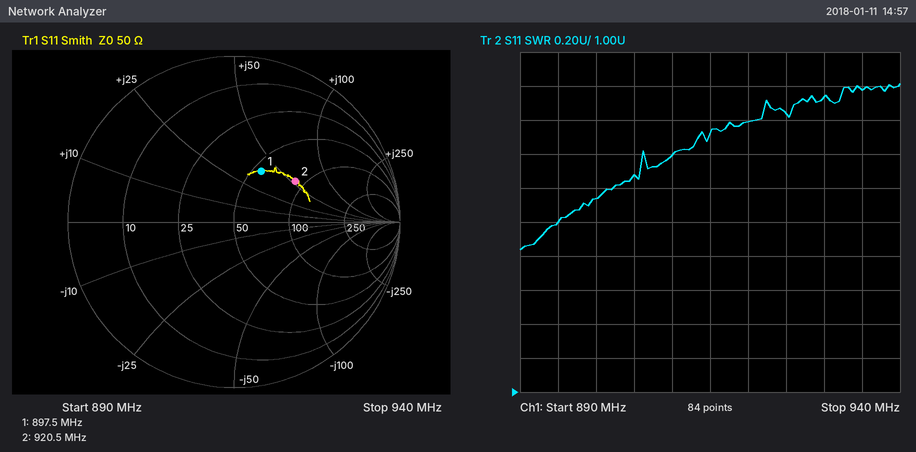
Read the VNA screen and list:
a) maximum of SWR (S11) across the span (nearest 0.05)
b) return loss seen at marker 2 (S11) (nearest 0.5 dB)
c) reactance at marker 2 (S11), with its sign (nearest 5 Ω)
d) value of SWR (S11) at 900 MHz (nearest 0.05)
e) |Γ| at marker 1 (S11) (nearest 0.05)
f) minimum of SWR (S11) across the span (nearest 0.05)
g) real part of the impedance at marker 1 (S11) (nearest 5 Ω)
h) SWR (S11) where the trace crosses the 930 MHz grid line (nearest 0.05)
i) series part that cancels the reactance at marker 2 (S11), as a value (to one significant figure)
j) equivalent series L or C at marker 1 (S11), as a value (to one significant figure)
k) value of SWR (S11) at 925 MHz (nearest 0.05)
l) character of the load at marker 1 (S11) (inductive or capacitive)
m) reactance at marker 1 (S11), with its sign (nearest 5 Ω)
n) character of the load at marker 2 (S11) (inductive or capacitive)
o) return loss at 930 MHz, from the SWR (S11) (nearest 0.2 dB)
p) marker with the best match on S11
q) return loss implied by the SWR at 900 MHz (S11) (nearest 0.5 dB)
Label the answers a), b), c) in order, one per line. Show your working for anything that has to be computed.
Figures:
a) 2.80
b) 7.0 dB
c) +55 Ω
d) 2.15
e) 0.35
f) 1.85
g) 55 Ω
h) 2.75
i) C = 1/(2π × 920.5 MHz × 55 Ω) ≈ 3 pF
j) L = 40 Ω/(2π × 897.5 MHz) ≈ 7 nH
k) 2.65
l) inductive
m) +40 Ω
n) inductive
o) −20 log10((2.75 − 1)/(2.75 + 1)) ≈ 6.6 dB
p) marker 1
q) −20 log10((2.15 − 1)/(2.15 + 1)) ≈ 8.75 dB, so 9.0 dB to the nearest 0.5 dB
